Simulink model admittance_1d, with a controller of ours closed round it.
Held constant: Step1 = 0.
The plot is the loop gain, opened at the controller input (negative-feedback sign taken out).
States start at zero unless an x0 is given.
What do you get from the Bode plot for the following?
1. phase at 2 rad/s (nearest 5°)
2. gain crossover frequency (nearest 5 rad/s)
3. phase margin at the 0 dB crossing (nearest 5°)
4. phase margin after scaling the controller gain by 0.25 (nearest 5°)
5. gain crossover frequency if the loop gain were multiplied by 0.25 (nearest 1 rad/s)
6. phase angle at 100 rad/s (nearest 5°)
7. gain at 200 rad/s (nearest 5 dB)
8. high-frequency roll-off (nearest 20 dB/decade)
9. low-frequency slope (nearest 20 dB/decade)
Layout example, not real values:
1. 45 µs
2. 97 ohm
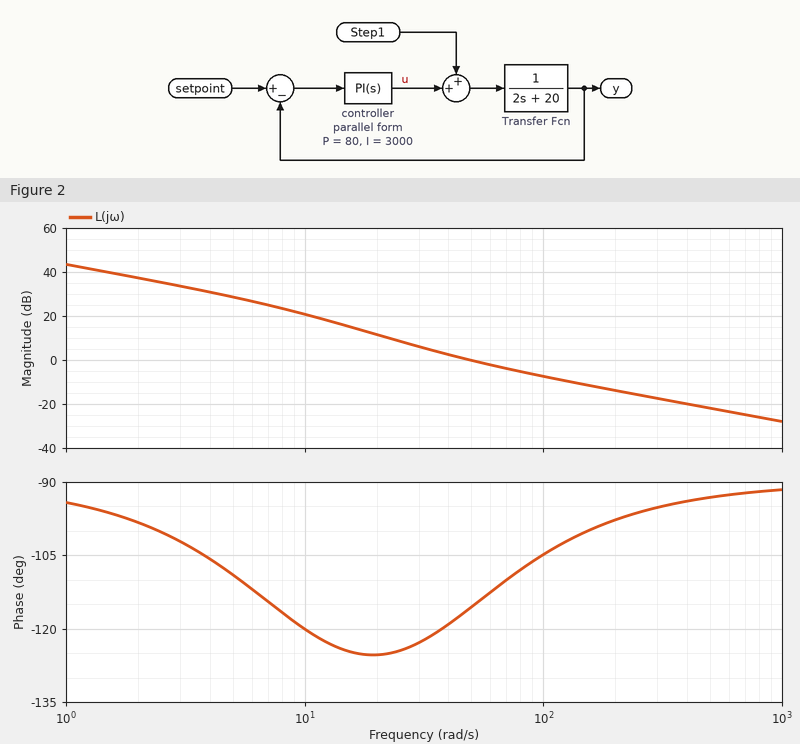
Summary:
1. -100°
2. 50 rad/s
3. 65°
4. 55°
5. 19 rad/s
6. -105°
7. -15 dB
8. -20 dB/decade
9. -20 dB/decade
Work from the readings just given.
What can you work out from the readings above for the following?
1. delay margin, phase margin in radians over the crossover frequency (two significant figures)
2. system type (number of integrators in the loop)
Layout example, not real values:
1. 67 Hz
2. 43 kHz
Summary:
1. 0.023 s
2. 1
